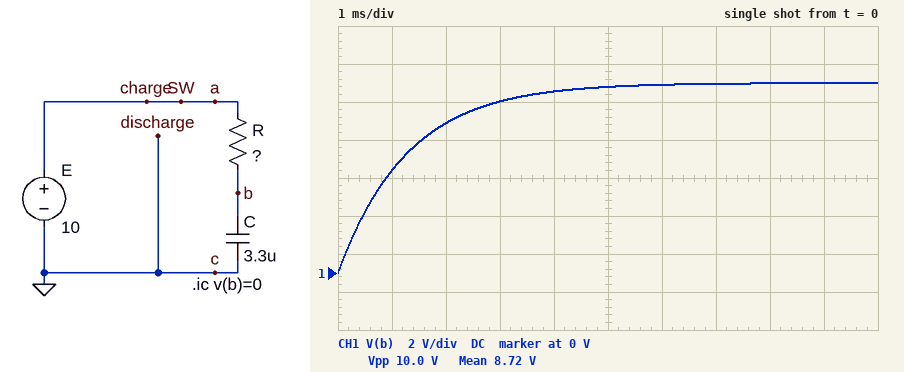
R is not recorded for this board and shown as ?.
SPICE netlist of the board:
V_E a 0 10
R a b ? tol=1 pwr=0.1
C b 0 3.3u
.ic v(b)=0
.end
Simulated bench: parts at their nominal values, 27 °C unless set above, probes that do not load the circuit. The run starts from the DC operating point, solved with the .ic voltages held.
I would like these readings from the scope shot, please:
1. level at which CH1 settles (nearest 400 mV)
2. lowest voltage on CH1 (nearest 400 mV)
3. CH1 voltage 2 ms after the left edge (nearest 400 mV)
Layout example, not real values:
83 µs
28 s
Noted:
10.0 V
0 V
8.0 V
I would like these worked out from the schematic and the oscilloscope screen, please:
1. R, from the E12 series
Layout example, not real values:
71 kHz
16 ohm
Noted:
390 Ω
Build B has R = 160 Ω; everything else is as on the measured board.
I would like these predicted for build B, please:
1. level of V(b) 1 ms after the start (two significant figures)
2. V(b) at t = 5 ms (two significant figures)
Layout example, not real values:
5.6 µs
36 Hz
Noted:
8.5 V
10 V
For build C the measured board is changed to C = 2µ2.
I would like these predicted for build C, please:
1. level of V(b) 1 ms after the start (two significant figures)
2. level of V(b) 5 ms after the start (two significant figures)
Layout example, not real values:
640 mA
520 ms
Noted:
6.9 V
10 V
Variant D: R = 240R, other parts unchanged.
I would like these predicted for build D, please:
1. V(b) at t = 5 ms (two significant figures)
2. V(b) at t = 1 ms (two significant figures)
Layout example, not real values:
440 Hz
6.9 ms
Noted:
10 V
7.2 V
